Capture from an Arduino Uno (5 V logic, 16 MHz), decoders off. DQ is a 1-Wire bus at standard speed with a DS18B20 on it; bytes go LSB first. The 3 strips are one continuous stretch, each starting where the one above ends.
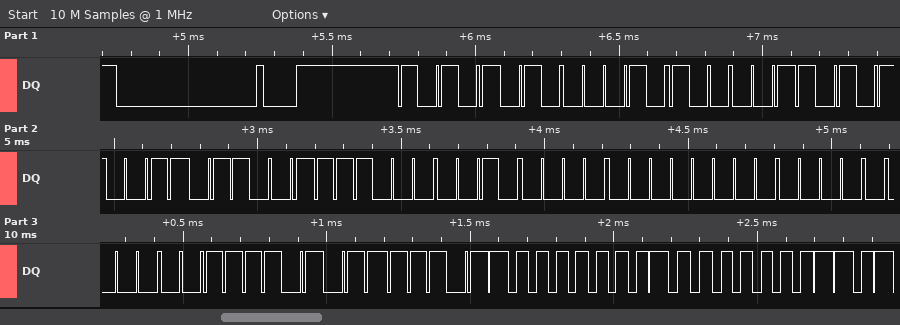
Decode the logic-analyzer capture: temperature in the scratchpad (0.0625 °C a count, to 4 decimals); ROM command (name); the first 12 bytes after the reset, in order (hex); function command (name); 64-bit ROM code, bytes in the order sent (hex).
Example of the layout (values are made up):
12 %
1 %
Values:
16.0625 °C
Match ROM
55 28 AC 6C 1E 04 00 00 BC BE 01 01
Read Scratchpad
28 AC 6C 1E 04 00 00 BC
